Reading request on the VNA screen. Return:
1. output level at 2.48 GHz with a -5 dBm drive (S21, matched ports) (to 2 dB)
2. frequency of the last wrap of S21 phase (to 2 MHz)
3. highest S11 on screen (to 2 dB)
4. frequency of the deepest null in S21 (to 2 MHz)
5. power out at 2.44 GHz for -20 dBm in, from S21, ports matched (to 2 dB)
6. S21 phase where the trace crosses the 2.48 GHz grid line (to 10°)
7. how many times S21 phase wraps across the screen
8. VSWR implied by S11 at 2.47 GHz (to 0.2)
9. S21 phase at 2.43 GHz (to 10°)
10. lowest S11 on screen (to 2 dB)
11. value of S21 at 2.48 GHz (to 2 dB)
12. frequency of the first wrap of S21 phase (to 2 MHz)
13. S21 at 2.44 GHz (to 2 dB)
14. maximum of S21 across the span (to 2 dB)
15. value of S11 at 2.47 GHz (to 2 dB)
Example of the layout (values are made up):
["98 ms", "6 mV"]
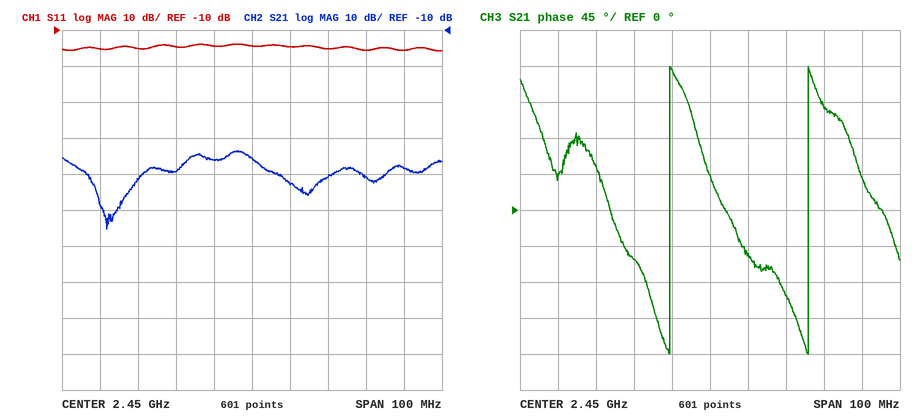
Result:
["-56 dBm", "2.476 GHz", "-14 dB", "2.412 GHz", "-66 dBm", "130°", "2", "1.4", "-60°", "-16 dB", "-50 dB", "2.440 GHz", "-46 dB", "-44 dB", "-16 dB"]
